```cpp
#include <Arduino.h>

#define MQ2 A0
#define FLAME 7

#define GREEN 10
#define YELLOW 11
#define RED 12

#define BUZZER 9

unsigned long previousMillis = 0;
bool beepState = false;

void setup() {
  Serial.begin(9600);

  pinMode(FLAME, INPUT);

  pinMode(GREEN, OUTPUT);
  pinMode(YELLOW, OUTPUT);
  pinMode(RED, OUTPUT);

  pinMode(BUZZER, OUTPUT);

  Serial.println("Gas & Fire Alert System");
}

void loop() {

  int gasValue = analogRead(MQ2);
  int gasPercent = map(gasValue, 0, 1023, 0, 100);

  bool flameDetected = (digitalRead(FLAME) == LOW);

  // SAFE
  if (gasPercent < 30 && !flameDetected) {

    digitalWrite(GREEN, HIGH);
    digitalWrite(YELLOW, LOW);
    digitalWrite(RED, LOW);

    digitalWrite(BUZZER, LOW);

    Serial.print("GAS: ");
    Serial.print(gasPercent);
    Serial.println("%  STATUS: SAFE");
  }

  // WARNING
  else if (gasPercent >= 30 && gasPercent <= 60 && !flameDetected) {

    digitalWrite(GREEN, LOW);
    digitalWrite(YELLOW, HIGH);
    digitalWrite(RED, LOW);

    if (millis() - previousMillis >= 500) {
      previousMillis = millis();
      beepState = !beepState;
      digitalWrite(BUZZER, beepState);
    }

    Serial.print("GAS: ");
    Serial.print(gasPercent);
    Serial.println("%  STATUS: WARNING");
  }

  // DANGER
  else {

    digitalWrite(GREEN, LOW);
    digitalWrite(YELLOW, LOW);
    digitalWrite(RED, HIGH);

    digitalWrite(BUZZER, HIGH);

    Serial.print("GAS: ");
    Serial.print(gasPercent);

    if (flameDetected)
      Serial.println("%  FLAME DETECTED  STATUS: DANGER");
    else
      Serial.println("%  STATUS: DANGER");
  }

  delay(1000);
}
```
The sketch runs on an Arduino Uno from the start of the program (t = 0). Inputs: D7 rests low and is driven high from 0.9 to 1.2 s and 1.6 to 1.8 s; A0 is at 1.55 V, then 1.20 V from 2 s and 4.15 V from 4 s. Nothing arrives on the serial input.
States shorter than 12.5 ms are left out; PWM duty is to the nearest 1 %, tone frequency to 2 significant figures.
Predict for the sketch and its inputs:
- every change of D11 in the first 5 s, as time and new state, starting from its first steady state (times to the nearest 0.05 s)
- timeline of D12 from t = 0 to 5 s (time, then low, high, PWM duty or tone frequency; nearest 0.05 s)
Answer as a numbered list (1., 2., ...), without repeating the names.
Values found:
1. 0 s low; 1 s high; 2 s low
2. 0 s high; 1 s low; 2 s high
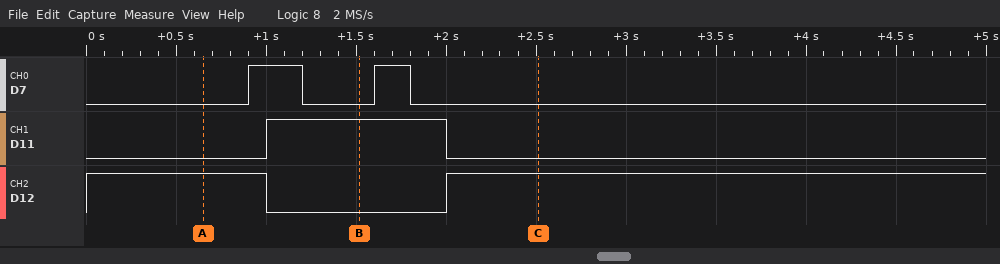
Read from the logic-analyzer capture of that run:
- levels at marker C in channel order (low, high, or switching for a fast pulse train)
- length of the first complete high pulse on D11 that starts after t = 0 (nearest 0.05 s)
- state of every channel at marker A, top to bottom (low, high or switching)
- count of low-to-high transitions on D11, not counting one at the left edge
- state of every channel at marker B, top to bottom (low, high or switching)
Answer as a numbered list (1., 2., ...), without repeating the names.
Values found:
1. D7 low, D11 low, D12 high
2. 1.00 s
3. D7 low, D11 low, D12 high
4. 1
5. D7 low, D11 high, D12 low
